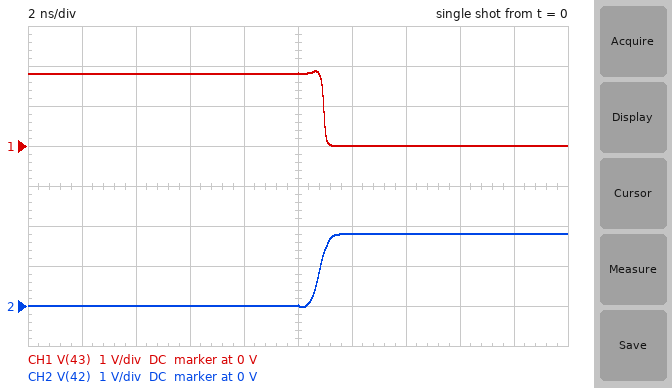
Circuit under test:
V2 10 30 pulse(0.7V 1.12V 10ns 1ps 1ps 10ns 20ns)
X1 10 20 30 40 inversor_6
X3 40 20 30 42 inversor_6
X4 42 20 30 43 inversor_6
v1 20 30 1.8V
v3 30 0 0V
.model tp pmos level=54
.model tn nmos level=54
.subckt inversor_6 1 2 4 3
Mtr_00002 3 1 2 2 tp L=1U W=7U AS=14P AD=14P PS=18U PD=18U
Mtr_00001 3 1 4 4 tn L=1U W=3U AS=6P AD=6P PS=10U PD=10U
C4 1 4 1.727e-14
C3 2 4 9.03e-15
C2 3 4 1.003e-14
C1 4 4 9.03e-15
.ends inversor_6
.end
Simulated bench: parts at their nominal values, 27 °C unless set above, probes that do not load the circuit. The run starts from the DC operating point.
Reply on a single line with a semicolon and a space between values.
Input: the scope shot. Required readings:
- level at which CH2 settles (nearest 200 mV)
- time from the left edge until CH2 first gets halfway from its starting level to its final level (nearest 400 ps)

1.8 V; 10.8 ns
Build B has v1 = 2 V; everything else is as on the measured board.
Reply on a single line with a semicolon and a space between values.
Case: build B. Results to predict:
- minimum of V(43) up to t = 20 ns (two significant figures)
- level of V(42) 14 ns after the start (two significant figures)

-22 mV; 2.0 V
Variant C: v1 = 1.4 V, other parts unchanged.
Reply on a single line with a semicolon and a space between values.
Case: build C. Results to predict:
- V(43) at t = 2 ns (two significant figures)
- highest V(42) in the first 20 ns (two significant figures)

24 mV; 1.4 V
